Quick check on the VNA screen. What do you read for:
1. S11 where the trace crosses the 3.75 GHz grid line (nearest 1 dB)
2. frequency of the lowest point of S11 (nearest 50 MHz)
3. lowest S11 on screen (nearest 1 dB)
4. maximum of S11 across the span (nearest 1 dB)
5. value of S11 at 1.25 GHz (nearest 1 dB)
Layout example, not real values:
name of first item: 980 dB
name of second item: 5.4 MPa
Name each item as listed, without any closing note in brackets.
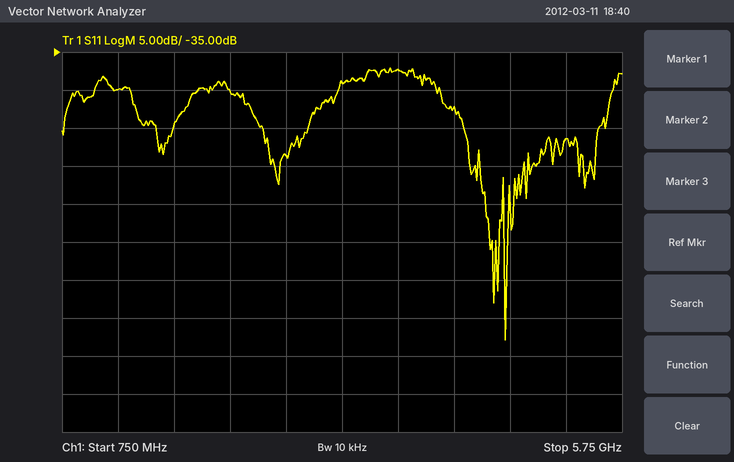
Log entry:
S11 where the trace crosses the 3.75 GHz grid line: -37 dB
frequency of the lowest point of S11: 4.70 GHz
lowest S11 on screen: -73 dB
maximum of S11 across the span: -37 dB
value of S11 at 1.25 GHz: -40 dB
